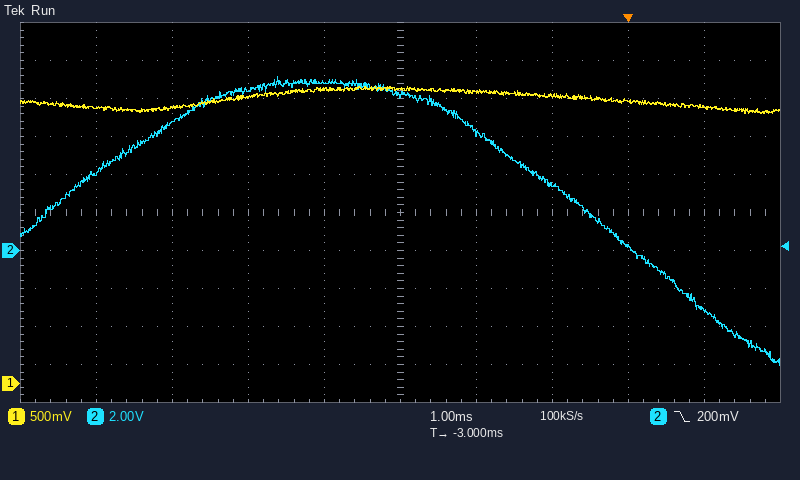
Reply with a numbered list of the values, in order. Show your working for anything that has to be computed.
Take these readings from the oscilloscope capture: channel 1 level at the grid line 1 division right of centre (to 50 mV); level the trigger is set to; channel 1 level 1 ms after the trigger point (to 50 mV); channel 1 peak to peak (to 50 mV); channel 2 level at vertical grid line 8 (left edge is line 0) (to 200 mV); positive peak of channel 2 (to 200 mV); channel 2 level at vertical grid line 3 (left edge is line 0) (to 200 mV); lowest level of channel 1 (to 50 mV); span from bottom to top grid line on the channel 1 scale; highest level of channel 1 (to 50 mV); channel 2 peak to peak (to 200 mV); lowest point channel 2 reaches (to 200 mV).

1. 3.85 V
2. 200 mV
3. 3.65 V
4. 3.90 V − (3.55 V) = 350 mV
5. 200 mV
6. 9.2 V
7. 8.4 V
8. 3.55 V
9. 5 V
10. 3.90 V
11. 9.2 V − (-6.0 V) = 15.2 V
12. -6.0 V
